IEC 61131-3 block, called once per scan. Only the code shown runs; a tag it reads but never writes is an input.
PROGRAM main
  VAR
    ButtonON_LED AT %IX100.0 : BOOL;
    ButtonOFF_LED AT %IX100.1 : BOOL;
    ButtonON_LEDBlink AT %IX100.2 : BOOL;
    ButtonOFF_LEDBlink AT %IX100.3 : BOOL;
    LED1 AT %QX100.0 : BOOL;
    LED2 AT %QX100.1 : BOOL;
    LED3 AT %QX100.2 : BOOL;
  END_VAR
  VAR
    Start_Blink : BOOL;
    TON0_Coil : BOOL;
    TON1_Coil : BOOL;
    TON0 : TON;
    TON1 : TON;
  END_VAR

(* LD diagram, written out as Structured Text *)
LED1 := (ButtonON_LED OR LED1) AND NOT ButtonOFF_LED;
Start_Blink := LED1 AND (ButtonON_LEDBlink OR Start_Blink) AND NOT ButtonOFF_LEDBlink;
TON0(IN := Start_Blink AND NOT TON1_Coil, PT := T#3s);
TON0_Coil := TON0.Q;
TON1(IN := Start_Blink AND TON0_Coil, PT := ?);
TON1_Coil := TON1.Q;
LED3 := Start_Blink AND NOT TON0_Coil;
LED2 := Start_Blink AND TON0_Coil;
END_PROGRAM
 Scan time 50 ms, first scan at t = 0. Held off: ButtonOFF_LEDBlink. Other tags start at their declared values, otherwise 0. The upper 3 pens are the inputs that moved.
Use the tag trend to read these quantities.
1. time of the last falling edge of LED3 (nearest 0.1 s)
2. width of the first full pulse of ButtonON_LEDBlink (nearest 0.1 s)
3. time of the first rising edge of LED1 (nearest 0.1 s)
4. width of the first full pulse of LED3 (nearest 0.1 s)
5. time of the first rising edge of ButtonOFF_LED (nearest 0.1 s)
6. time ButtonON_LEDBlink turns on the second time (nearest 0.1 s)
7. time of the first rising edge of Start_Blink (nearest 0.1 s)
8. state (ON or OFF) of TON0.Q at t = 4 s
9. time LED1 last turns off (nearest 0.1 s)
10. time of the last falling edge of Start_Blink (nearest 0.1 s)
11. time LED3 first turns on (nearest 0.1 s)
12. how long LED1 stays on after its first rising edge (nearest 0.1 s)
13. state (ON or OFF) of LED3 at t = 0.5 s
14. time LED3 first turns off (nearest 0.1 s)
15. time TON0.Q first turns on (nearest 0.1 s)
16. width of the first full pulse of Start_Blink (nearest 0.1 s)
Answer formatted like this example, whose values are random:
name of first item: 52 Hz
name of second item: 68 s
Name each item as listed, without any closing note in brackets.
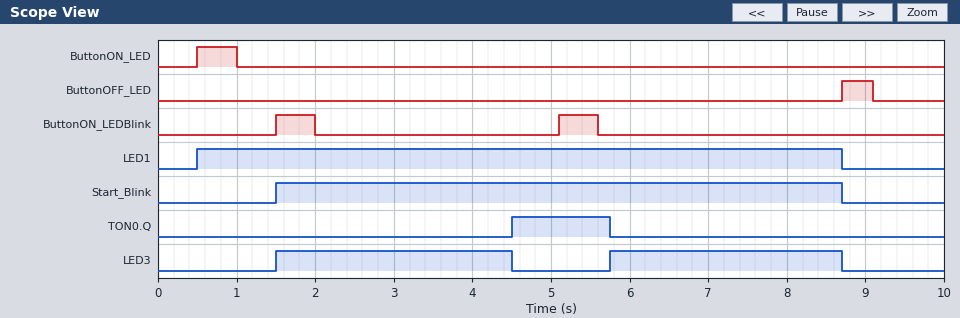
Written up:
time of the last falling edge of LED3: 8.7 s
width of the first full pulse of ButtonON_LEDBlink: 0.5 s
time of the first rising edge of LED1: 0.5 s
width of the first full pulse of LED3: 3.0 s
time of the first rising edge of ButtonOFF_LED: 8.7 s
time ButtonON_LEDBlink turns on the second time: 5.1 s
time of the first rising edge of Start_Blink: 1.5 s
state (ON or OFF) of TON0.Q at t = 4 s: OFF
time LED1 last turns off: 8.7 s
time of the last falling edge of Start_Blink: 8.7 s
time LED3 first turns on: 1.5 s
how long LED1 stays on after its first rising edge: 8.2 s
state (ON or OFF) of LED3 at t = 0.5 s: OFF
time LED3 first turns off: 4.5 s
time TON0.Q first turns on: 4.5 s
width of the first full pulse of Start_Blink: 7.2 s
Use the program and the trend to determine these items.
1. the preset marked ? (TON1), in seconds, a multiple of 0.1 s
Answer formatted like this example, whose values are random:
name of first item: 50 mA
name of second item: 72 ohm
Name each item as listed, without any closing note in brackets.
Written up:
the preset marked ? (TON1), in seconds, a multiple of 0.1 s: 1.2 s
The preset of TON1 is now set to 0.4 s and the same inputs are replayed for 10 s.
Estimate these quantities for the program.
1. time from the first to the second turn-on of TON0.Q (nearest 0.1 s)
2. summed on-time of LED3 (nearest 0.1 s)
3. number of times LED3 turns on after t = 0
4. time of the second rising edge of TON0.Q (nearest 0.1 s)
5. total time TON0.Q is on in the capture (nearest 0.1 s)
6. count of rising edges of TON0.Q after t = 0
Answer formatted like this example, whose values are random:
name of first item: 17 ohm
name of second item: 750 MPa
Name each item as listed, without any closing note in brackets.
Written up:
time from the first to the second turn-on of TON0.Q: 3.5 s
summed on-time of LED3: 6.3 s
number of times LED3 turns on after t = 0: 3
time of the second rising edge of TON0.Q: 8.0 s
total time TON0.Q is on in the capture: 0.9 s
count of rising edges of TON0.Q after t = 0: 2
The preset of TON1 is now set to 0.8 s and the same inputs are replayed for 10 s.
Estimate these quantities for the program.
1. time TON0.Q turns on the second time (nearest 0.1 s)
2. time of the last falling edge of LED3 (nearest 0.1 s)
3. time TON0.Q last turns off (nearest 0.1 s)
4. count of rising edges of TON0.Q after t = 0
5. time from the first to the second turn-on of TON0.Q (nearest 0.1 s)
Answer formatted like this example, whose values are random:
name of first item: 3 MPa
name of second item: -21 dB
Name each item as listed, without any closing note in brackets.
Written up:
time TON0.Q turns on the second time: 8.4 s
time of the last falling edge of LED3: 8.4 s
time TON0.Q last turns off: 8.7 s
count of rising edges of TON0.Q after t = 0: 2
time from the first to the second turn-on of TON0.Q: 3.9 s
